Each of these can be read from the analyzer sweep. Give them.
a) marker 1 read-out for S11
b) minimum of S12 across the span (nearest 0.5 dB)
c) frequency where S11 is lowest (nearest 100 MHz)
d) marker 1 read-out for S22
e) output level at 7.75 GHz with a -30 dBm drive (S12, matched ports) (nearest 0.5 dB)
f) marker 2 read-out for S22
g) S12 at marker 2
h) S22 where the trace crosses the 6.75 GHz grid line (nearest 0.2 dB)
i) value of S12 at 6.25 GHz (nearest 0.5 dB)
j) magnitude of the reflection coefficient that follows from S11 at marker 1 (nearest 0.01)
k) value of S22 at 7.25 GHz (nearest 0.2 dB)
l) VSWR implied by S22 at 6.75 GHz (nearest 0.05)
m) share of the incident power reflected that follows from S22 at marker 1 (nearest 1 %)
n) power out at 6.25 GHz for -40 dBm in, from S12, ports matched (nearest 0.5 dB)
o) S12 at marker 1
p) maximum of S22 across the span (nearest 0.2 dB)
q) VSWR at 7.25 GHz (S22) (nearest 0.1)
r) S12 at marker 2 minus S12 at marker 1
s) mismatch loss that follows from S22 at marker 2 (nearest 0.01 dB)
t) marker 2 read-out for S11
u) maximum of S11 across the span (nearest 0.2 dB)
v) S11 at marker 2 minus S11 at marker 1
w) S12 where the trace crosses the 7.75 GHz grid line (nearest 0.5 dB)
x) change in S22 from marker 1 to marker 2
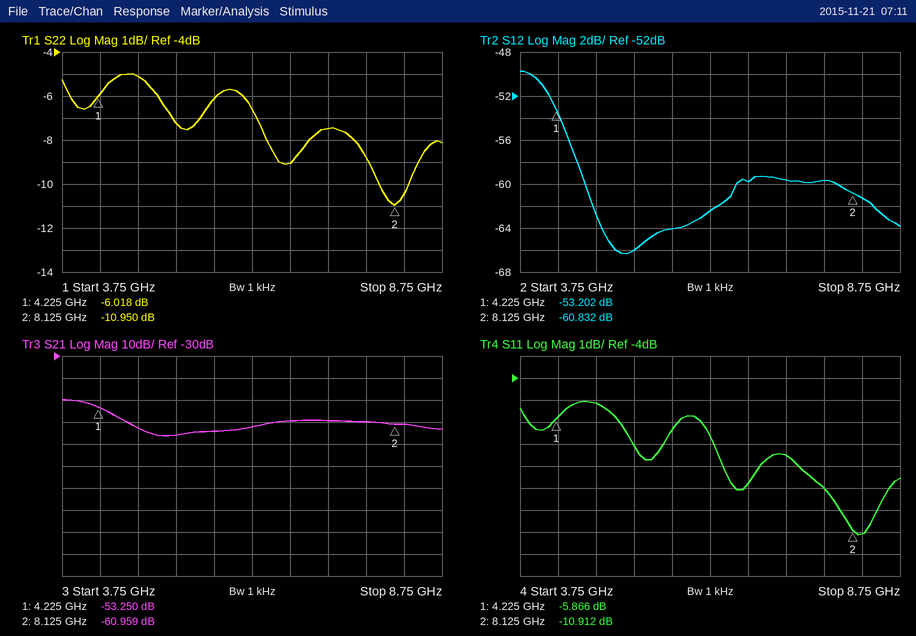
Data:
-5.866 dB
-66.5 dB
8.2 GHz
-6.018 dB
-89.5 dBm
-10.950 dB
-60.832 dB
-9.0 dB
-62.5 dB
0.51
-7.4 dB
2.10
25 %
-102.5 dBm
-53.202 dB
-5.0 dB
2.5
-7.630 dB
0.36 dB
-10.912 dB
-5.0 dB
-5.046 dB
-59.5 dB
-4.932 dB
